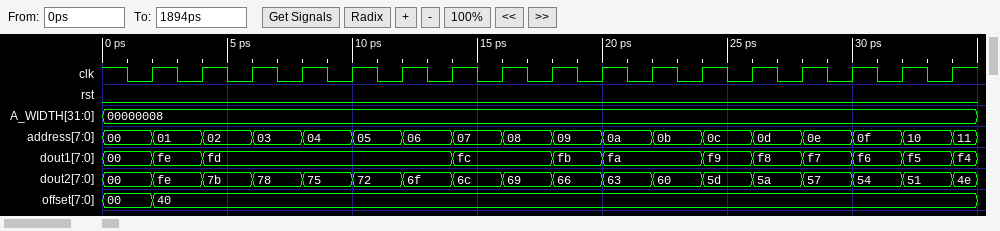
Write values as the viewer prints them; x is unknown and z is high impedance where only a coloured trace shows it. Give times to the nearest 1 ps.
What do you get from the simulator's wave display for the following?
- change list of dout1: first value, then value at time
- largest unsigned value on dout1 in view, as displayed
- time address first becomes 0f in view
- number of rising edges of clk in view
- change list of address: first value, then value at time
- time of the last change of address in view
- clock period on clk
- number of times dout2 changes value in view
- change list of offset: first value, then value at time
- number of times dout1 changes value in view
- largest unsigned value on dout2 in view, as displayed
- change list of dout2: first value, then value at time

00, fe at 2 ps, fd at 4 ps, fc at 14 ps, fb at 18 ps, fa at 20 ps, f9 at 24 ps, f8 at 26 ps, f7 at 28 ps, f6 at 30 ps, f5 at 32 ps, f4 at 34 ps
fe
30 ps
17
00, 01 at 2 ps, 02 at 4 ps, 03 at 6 ps, 04 at 8 ps, 05 at 10 ps, 06 at 12 ps, 07 at 14 ps, 08 at 16 ps, 09 at 18 ps, 0a at 20 ps, 0b at 22 ps, 0c at 24 ps, 0d at 26 ps, 0e at 28 ps, 0f at 30 ps, 10 at 32 ps, 11 at 34 ps
34 ps
2 ps
17
00, 40 at 2 ps
11
fe
00, fe at 2 ps, 7b at 4 ps, 78 at 6 ps, 75 at 8 ps, 72 at 10 ps, 6f at 12 ps, 6c at 14 ps, 69 at 16 ps, 66 at 18 ps, 63 at 20 ps, 60 at 22 ps, 5d at 24 ps, 5a at 26 ps, 57 at 28 ps, 54 at 30 ps, 51 at 32 ps, 4e at 34 ps
